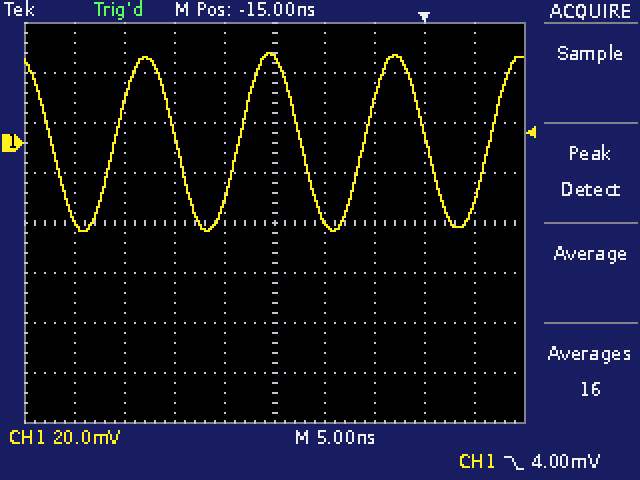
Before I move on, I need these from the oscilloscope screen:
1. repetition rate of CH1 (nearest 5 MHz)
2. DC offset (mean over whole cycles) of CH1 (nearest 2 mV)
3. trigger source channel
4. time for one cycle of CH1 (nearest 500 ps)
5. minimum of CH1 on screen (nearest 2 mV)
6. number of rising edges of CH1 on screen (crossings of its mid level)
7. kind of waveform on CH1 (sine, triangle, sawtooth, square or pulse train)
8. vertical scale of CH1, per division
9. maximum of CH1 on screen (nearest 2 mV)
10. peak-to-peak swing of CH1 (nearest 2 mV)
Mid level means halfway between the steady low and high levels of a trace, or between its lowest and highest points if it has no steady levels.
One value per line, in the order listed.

80 MHz
0 mV
CH1
12.5 ns
-36 mV
4
sine
20 mV
36 mV
72 mV
